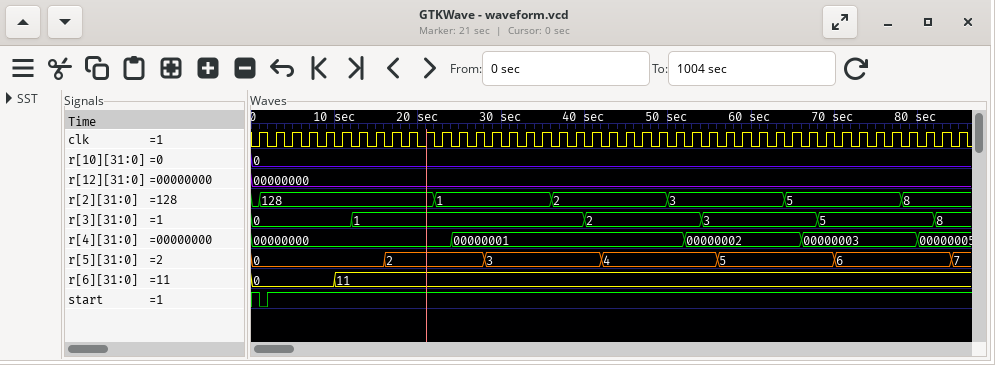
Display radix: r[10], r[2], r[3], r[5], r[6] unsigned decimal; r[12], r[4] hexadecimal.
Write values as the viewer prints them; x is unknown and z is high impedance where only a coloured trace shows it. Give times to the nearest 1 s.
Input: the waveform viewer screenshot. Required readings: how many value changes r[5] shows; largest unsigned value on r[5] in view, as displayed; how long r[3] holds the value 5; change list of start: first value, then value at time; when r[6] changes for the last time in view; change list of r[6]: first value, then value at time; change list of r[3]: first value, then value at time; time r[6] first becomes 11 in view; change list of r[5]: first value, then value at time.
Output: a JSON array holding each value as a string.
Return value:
["6", "7", "14 s", "1, 0 at 1 s, 1 at 2 s", "10 s", "0, 11 at 10 s", "0, 1 at 12 s, 2 at 40 s, 3 at 54 s, 5 at 68 s, 8 at 82 s", "10 s", "0, 2 at 16 s, 3 at 28 s, 4 at 42 s, 5 at 56 s, 6 at 70 s, 7 at 84 s"]
